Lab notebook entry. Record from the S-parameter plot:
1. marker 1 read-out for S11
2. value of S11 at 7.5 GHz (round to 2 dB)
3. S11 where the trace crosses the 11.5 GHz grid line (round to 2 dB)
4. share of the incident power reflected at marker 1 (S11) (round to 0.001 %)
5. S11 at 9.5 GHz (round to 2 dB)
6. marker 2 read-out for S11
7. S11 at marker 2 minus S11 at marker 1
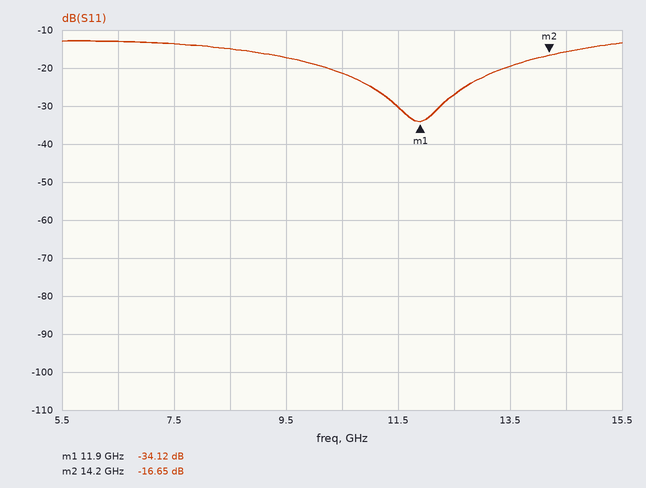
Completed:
-34.12 dB
-14 dB
-30 dB
0.039 %
-18 dB
-16.65 dB
17.47 dB
